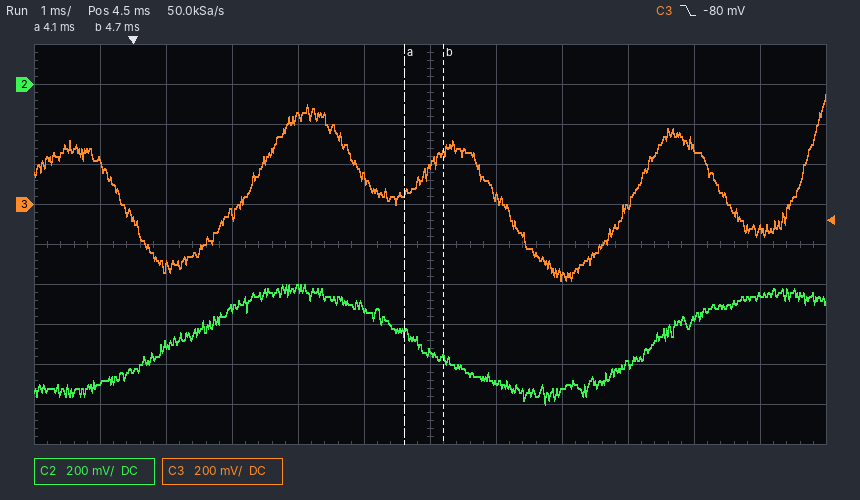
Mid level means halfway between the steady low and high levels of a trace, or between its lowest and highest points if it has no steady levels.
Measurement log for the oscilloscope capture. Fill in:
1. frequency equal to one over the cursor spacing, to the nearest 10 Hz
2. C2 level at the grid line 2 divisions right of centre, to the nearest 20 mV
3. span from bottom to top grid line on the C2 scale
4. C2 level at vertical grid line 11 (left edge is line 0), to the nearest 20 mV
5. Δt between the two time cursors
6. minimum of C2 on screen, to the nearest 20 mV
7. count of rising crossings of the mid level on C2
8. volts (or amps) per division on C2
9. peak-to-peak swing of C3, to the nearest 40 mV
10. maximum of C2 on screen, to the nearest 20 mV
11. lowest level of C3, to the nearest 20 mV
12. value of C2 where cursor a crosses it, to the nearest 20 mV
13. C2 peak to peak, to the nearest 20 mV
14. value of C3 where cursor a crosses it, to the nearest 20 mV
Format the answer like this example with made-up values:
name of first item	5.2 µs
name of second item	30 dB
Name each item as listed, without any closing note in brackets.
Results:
frequency equal to one over the cursor spacing, to the nearest 10 Hz	1.67 kHz
C2 level at the grid line 2 divisions right of centre, to the nearest 20 mV	-1.54 V
span from bottom to top grid line on the C2 scale	2 V
C2 level at vertical grid line 11 (left edge is line 0), to the nearest 20 mV	-1.06 V
Δt between the two time cursors	600 µs
minimum of C2 on screen, to the nearest 20 mV	-1.60 V
count of rising crossings of the mid level on C2	2
volts (or amps) per division on C2	200 mV
peak-to-peak swing of C3, to the nearest 40 mV	920 mV
maximum of C2 on screen, to the nearest 20 mV	-1.00 V
lowest level of C3, to the nearest 20 mV	-380 mV
value of C2 where cursor a crosses it, to the nearest 20 mV	-1.24 V
C2 peak to peak, to the nearest 20 mV	600 mV
value of C3 where cursor a crosses it, to the nearest 20 mV	60 mV
